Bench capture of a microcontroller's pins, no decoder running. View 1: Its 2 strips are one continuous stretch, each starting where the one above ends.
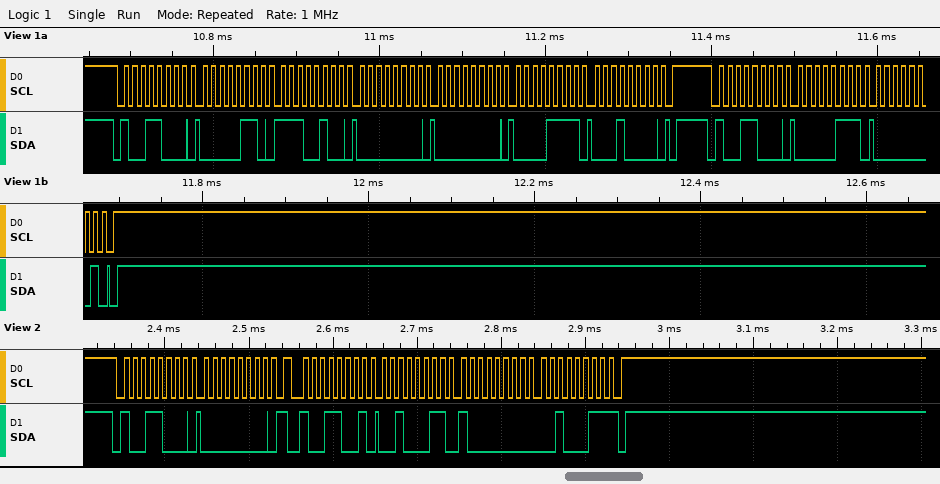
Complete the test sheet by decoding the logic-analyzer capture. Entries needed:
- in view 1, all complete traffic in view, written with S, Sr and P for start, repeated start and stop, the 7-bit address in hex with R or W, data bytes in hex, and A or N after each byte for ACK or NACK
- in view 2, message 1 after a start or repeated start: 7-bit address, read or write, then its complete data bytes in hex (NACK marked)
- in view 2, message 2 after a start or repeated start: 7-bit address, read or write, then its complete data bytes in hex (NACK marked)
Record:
S 4CW A 06 A E4 A 00 A 00 A 0F A 10 A P S 4CW A 07 A 01 A P
0x4C write: 00
0x4C read: 23 80 23 NACK
